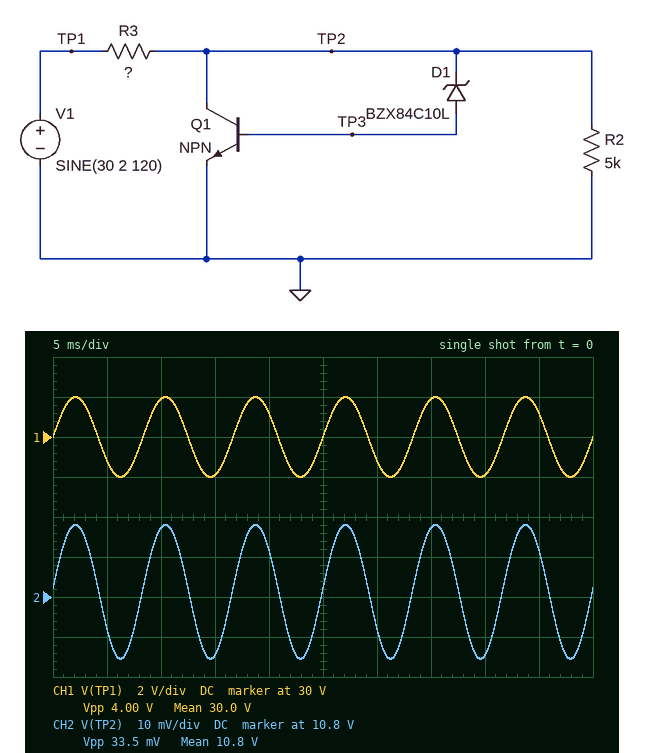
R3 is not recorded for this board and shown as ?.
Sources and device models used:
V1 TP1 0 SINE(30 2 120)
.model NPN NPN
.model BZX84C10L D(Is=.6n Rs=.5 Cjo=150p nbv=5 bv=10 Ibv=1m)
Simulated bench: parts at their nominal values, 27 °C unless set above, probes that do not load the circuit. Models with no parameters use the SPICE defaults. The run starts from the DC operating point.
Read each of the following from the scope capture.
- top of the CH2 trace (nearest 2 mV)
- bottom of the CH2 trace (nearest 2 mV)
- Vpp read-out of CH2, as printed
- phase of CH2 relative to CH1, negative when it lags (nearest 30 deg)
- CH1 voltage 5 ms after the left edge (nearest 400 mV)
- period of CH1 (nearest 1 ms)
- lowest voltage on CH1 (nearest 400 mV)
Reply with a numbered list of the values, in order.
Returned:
1. 10.818 V
2. 10.784 V
3. 33.5 mV
4. 0 deg
5. 28.8 V
6. 8 ms
7. 28.0 V
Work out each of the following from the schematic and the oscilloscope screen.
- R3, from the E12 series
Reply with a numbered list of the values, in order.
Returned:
1. 330 Ω
